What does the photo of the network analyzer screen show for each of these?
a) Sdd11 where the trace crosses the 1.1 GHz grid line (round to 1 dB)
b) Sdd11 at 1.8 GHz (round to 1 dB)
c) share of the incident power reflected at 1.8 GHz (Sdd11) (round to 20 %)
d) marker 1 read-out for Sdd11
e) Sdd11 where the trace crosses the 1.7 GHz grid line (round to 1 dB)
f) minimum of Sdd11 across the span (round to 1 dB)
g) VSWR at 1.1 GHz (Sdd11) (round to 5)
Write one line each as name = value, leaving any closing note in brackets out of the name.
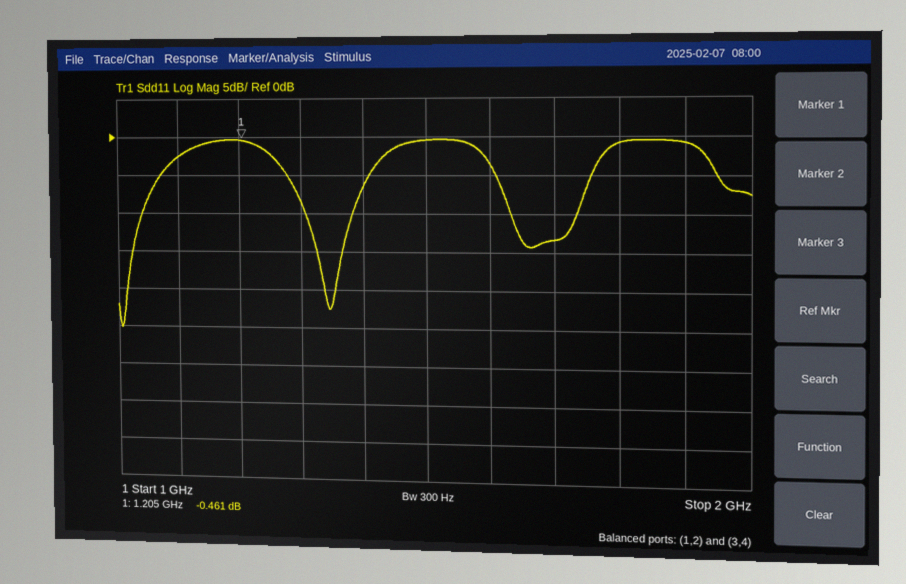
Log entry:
Sdd11 where the trace crosses the 1.1 GHz grid line = -3 dB
Sdd11 at 1.8 GHz = -1 dB
share of the incident power reflected at 1.8 GHz (Sdd11) = 80 %
marker 1 read-out for Sdd11 = -0.461 dB
Sdd11 where the trace crosses the 1.7 GHz grid line = -13 dB
minimum of Sdd11 across the span = -25 dB
VSWR at 1.1 GHz (Sdd11) = 5
